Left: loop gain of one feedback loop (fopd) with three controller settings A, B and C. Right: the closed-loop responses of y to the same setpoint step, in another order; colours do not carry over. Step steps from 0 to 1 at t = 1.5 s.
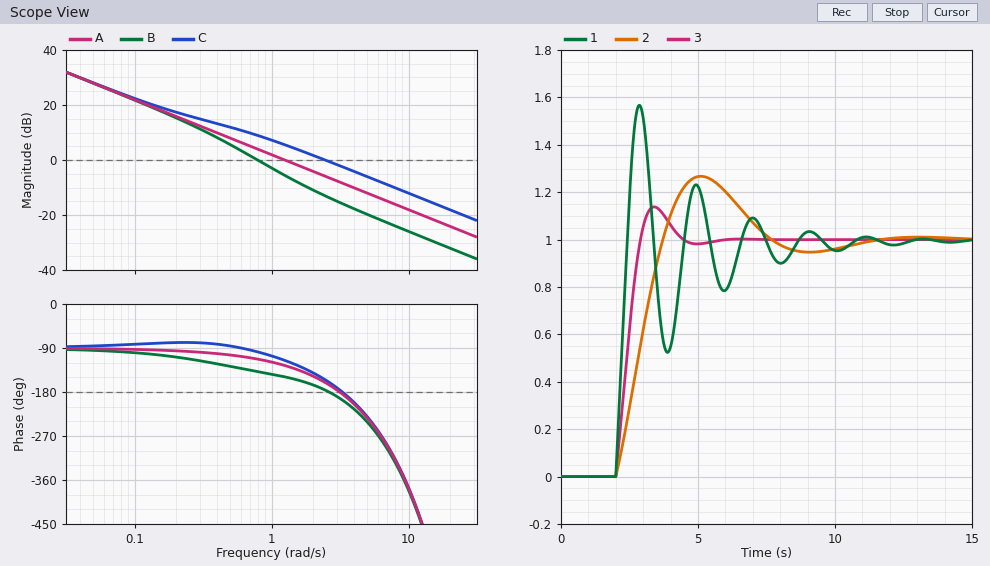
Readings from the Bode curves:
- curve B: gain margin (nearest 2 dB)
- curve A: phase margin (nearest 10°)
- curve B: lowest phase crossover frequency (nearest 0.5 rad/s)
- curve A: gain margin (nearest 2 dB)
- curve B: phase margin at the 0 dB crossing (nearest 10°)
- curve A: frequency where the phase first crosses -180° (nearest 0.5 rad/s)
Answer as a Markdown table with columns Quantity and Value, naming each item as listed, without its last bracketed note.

| Quantity | Value |
|---|---|
| curve B: gain margin | 14 dB |
| curve A: phase margin | 50° |
| curve B: lowest phase crossover frequency | 2.5 rad/s |
| curve A: gain margin | 8 dB |
| curve B: phase margin at the 0 dB crossing | 40° |
| curve A: frequency where the phase first crosses -180° | 3.0 rad/s |
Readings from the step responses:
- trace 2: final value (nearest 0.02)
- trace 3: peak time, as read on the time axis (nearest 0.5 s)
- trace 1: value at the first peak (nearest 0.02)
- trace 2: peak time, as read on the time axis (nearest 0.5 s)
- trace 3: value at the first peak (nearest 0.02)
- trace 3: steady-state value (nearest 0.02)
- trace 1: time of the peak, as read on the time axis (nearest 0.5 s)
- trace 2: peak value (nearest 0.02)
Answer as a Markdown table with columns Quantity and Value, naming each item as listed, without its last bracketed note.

| Quantity | Value |
|---|---|
| trace 2: final value | 1.00 |
| trace 3: peak time, as read on the time axis | 3.5 s |
| trace 1: value at the first peak | 1.56 |
| trace 2: peak time, as read on the time axis | 5.0 s |
| trace 3: value at the first peak | 1.14 |
| trace 3: steady-state value | 1.00 |
| trace 1: time of the peak, as read on the time axis | 3.0 s |
| trace 2: peak value | 1.26 |
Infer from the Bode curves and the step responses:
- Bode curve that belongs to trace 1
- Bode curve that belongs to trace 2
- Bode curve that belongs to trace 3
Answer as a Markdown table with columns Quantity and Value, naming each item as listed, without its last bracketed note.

| Quantity | Value |
|---|---|
| Bode curve that belongs to trace 1 | C |
| Bode curve that belongs to trace 2 | B |
| Bode curve that belongs to trace 3 | A |
